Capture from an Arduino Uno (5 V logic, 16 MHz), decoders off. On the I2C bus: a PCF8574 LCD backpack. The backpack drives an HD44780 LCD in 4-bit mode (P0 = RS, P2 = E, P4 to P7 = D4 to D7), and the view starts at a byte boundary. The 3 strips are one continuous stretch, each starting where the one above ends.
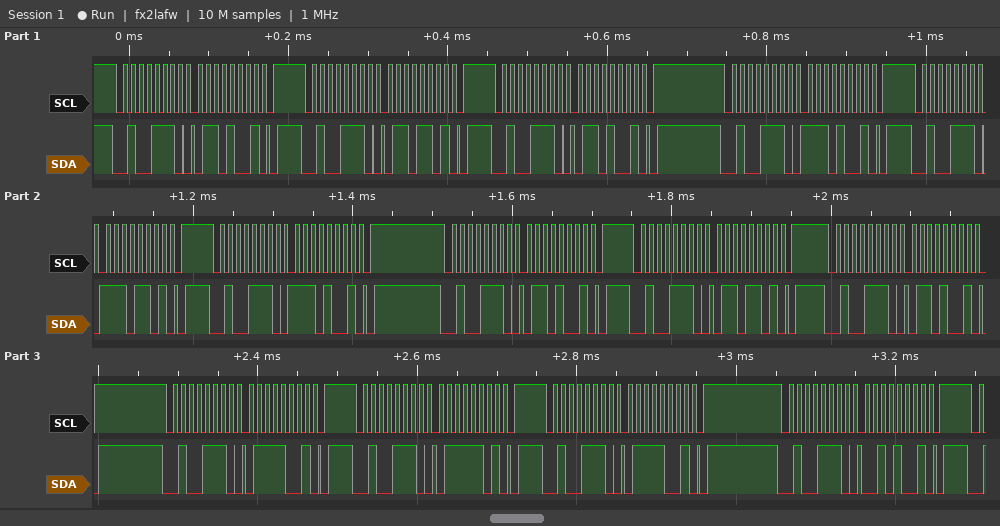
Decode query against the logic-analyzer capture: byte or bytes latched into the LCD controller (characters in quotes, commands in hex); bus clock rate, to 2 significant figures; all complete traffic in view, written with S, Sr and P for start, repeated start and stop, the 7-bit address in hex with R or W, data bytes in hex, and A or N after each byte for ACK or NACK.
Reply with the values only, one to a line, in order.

'n' 'g'
100 kHz
S 27W A 69 A P S 27W A 6D A P S 27W A 69 A P S 27W A E9 A P S 27W A ED A P S 27W A E9 A P S 27W A 69 A P S 27W A 6D A P S 27W A 69 A P S 27W A 79 A P S 27W A 7D A P S 27W A 79 A P S 27W A 29 A P
